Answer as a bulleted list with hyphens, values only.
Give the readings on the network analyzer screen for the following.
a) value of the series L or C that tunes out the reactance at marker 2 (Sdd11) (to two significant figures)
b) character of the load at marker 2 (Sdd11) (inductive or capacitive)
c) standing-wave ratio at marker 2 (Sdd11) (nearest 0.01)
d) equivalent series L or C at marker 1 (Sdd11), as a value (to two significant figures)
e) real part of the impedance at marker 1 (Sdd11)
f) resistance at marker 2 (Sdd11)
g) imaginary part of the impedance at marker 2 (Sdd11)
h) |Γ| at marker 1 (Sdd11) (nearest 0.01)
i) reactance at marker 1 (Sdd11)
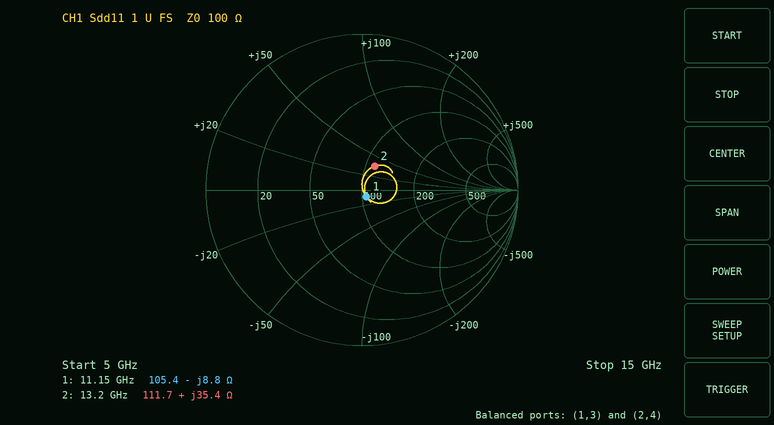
- 340 fF
- inductive
- 1.42
- 1.6 pF
- 105.4 Ω
- 111.7 Ω
- +35.4 Ω
- 0.05
- -8.8 Ω
